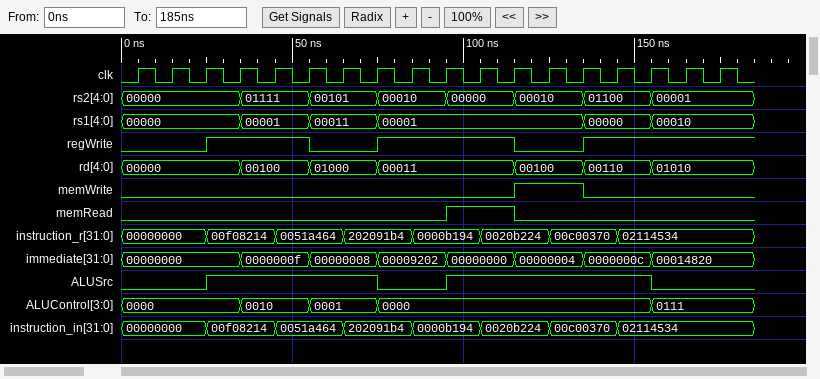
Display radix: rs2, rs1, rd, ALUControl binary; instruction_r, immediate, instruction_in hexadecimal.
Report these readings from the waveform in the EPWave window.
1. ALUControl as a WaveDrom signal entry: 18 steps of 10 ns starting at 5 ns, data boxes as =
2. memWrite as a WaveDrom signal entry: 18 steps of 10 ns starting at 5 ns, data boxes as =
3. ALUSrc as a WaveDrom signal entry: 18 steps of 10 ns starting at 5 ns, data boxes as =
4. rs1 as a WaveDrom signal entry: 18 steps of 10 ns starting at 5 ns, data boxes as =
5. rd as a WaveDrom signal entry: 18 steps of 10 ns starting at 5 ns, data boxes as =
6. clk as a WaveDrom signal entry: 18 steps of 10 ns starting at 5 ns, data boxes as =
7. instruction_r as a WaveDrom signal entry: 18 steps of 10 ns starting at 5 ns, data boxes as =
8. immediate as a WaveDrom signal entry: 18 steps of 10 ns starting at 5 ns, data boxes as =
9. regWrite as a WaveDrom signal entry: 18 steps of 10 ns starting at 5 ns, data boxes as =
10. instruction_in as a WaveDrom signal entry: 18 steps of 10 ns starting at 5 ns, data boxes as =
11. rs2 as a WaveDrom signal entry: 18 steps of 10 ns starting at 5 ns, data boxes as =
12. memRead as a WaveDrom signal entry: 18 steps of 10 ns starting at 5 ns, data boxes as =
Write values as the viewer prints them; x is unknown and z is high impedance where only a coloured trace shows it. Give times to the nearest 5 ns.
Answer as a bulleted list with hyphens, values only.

- {name: 'ALUControl', wave: '=..=.=.=.......=..', data: '0000 0010 0001 0000 0111'}
- {name: 'memWrite', wave: '0..........1.0....'}
- {name: 'ALUSrc', wave: '0.1....0.1.....0..'}
- {name: 'rs1', wave: '=..=.=.=.....=.=..', data: '00000 00001 00011 00001 00000 00010'}
- {name: 'rd', wave: '=..=.=.=...=.=.=..', data: '00000 00100 01000 00011 00100 00110 01010'}
- {name: 'clk', wave: 'p.................'}
- {name: 'instruction_r', wave: '=.=.=.=.=.=.=.=...', data: '00000000 00f08214 0051a464 202091b4 0000b194 0020b224 00c00370 02114534'}
- {name: 'immediate', wave: '=..=.=.=.=.=.=.=..', data: '00000000 0000000f 00000008 00009202 00000000 00000004 0000000c 00014820'}
- {name: 'regWrite', wave: '0.1..0.1...0.1....'}
- {name: 'instruction_in', wave: '=.=.=.=.=.=.=.=...', data: '00000000 00f08214 0051a464 202091b4 0000b194 0020b224 00c00370 02114534'}
- {name: 'rs2', wave: '=..=.=.=.=.=.=.=..', data: '00000 01111 00101 00010 00000 00010 01100 00001'}
- {name: 'memRead', wave: '0........1.0......'}
